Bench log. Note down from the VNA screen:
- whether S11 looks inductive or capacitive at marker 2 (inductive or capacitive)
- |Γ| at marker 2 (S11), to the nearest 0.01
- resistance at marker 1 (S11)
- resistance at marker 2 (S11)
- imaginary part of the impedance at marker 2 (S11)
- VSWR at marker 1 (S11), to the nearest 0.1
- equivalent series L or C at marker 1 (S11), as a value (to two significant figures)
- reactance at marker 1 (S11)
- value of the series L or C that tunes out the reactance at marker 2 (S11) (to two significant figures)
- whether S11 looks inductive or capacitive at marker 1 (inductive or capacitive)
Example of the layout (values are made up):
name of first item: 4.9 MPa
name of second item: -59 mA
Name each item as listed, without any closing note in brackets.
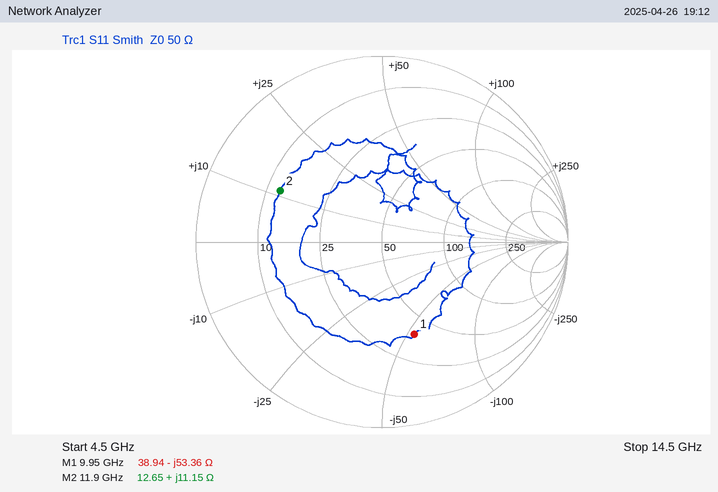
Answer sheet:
whether S11 looks inductive or capacitive at marker 2: inductive
|Γ| at marker 2 (S11), to the nearest 0.01: 0.61
resistance at marker 1: 38.94 Ω
resistance at marker 2: 12.65 Ω
imaginary part of the impedance at marker 2: +11.15 Ω
VSWR at marker 1 (S11), to the nearest 0.1: 3.2
equivalent series L or C at marker 1 (S11), as a value: 300 fF
reactance at marker 1: -53.36 Ω
value of the series L or C that tunes out the reactance at marker 2 (S11): 1.2 pF
whether S11 looks inductive or capacitive at marker 1: capacitive
